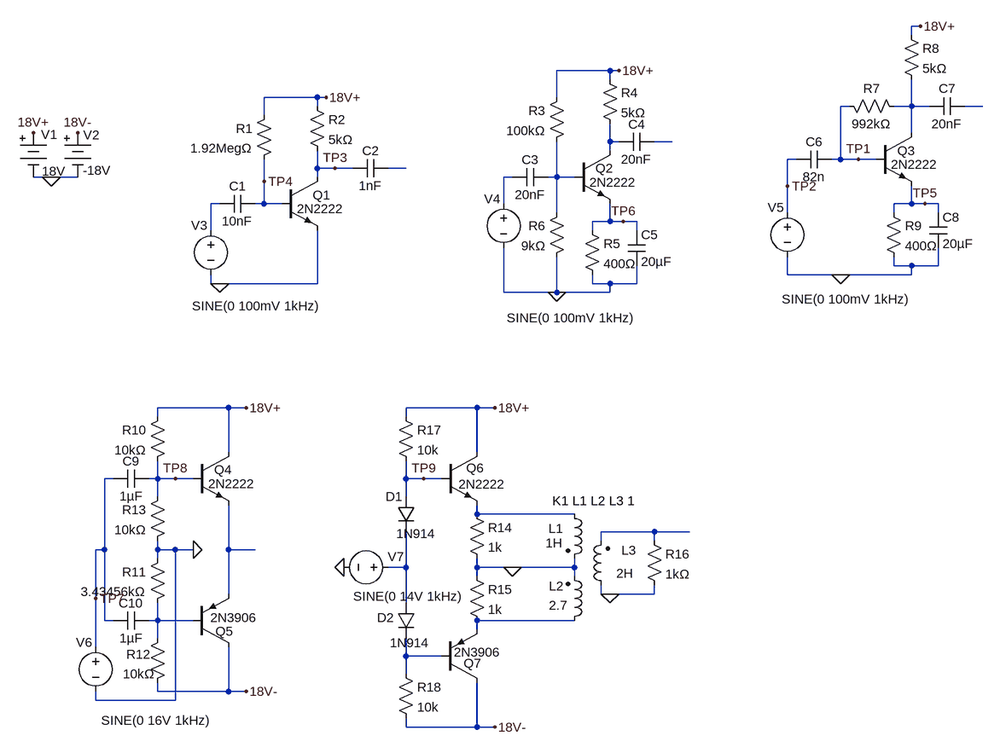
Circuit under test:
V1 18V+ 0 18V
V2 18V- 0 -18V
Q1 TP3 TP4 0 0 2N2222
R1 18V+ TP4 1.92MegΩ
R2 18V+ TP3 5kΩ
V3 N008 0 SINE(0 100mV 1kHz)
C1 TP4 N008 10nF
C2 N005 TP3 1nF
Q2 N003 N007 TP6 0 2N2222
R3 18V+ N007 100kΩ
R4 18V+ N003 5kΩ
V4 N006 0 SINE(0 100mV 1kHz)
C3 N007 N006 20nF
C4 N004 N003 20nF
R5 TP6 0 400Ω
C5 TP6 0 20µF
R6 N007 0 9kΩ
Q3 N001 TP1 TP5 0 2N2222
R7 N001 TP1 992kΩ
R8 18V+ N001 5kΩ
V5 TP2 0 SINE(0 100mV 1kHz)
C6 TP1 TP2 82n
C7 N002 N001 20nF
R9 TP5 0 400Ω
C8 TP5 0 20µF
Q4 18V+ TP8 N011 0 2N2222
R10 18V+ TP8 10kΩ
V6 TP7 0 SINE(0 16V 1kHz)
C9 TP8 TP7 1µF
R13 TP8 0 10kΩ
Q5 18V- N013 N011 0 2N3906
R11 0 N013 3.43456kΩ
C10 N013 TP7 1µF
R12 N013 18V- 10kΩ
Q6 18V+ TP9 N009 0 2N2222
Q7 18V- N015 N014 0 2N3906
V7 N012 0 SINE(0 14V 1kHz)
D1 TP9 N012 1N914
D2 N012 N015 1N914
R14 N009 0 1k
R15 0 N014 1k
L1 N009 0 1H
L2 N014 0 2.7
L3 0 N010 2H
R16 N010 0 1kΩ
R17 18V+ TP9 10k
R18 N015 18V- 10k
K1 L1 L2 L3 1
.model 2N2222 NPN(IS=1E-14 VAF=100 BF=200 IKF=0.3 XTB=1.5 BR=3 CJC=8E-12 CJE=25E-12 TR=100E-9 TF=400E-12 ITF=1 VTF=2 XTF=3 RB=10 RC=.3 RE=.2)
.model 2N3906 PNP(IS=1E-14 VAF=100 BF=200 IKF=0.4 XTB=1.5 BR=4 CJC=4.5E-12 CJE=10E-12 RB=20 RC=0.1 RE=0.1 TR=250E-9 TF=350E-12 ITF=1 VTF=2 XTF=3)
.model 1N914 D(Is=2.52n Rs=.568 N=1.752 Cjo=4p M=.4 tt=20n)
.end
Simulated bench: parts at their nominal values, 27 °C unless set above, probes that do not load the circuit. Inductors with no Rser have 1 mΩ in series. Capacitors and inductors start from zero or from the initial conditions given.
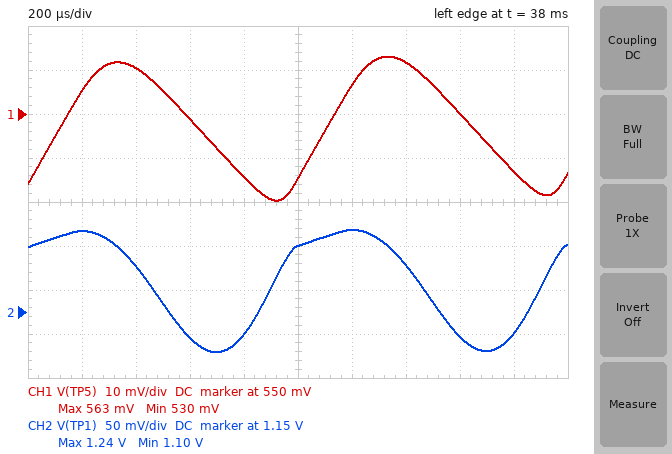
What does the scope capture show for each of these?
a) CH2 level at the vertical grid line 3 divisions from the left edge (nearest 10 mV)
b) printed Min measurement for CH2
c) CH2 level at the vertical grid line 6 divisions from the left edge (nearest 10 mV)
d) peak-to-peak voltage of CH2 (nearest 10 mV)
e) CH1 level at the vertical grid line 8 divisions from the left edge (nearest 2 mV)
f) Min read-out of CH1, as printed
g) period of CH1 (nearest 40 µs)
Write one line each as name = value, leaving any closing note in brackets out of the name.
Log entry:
CH2 level at the vertical grid line 3 divisions from the left edge = 1.12 V
printed Min measurement for CH2 = 1.10 V
CH2 level at the vertical grid line 6 divisions from the left edge = 1.24 V
peak-to-peak voltage of CH2 = 140 mV
CH1 level at the vertical grid line 8 divisions from the left edge = 550 mV
Min read-out of CH1, as printed = 530 mV
period of CH1 = 1.00 ms
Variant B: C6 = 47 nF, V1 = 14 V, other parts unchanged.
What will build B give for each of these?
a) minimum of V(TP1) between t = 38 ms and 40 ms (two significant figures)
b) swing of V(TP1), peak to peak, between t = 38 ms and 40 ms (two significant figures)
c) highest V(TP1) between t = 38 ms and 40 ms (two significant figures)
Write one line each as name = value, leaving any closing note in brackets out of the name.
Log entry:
minimum of V(TP1) between t = 38 ms and 40 ms = 1.0 V
swing of V(TP1), peak to peak, between t = 38 ms and 40 ms = 120 mV
highest V(TP1) between t = 38 ms and 40 ms = 1.1 V
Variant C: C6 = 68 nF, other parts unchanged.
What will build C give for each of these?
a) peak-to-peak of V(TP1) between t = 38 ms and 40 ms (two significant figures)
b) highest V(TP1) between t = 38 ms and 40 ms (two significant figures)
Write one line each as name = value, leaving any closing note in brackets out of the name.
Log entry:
peak-to-peak of V(TP1) between t = 38 ms and 40 ms = 130 mV
highest V(TP1) between t = 38 ms and 40 ms = 1.3 V
